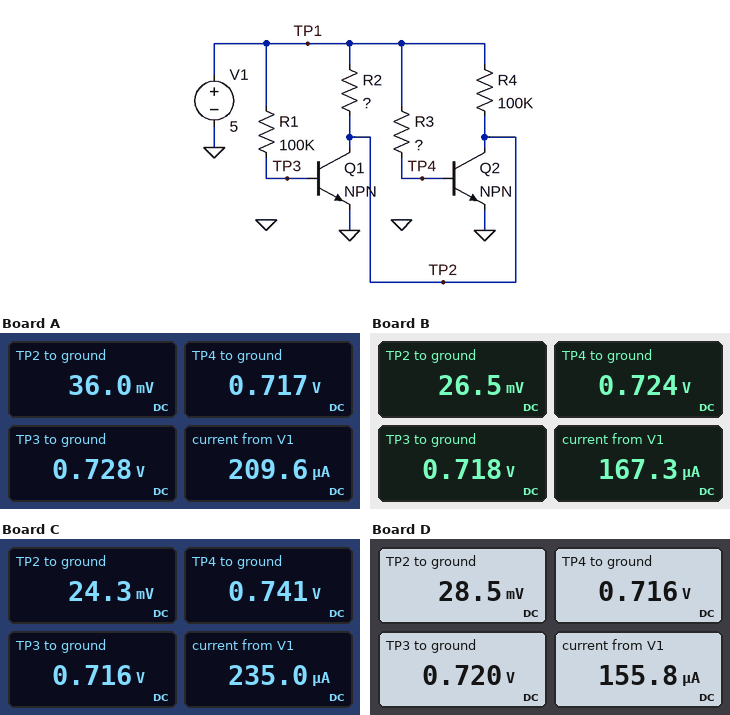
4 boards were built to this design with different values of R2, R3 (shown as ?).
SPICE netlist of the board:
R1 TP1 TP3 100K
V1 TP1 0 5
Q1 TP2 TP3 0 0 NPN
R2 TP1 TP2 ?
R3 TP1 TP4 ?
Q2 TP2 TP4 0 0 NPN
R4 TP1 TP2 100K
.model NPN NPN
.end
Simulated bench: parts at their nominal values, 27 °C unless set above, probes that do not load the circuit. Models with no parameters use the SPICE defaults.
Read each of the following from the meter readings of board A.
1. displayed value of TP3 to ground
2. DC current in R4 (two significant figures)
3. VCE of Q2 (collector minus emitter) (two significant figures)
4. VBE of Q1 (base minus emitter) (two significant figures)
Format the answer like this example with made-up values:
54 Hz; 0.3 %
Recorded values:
0.728 V; 50 µA; 36 mV; 730 mV
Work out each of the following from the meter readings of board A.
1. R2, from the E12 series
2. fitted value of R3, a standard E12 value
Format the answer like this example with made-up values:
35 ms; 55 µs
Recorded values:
56 kΩ; 150 kΩ
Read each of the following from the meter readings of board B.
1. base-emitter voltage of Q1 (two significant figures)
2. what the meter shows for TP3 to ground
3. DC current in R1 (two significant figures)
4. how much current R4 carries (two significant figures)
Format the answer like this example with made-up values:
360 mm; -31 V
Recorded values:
720 mV; 0.718 V; 43 µA; 50 µA
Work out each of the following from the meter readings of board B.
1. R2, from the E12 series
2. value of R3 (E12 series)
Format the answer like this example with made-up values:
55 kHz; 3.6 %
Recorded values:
220 kΩ; 82 kΩ
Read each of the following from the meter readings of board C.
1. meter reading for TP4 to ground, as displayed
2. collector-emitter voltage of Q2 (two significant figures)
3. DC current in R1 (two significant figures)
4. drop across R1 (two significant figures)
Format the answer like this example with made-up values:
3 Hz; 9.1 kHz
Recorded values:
0.741 V; 24 mV; 43 µA; 4.3 V
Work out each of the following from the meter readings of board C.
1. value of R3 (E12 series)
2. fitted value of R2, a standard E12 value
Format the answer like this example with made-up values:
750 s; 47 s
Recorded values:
39 kΩ; 150 kΩ
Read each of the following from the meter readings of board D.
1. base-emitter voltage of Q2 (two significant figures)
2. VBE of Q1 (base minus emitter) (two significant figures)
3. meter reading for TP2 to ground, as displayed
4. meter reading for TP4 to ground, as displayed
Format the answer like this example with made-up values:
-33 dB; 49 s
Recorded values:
720 mV; 720 mV; 28.5 mV; 0.716 V
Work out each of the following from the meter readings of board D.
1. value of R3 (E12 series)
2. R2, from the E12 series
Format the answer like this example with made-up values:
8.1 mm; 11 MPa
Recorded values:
120 kΩ; 180 kΩ
